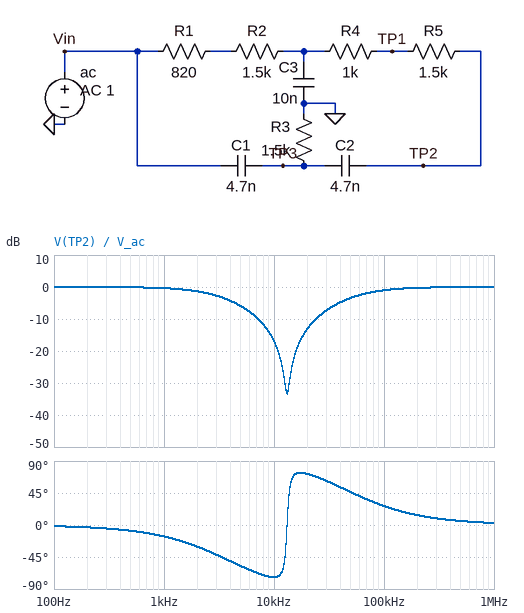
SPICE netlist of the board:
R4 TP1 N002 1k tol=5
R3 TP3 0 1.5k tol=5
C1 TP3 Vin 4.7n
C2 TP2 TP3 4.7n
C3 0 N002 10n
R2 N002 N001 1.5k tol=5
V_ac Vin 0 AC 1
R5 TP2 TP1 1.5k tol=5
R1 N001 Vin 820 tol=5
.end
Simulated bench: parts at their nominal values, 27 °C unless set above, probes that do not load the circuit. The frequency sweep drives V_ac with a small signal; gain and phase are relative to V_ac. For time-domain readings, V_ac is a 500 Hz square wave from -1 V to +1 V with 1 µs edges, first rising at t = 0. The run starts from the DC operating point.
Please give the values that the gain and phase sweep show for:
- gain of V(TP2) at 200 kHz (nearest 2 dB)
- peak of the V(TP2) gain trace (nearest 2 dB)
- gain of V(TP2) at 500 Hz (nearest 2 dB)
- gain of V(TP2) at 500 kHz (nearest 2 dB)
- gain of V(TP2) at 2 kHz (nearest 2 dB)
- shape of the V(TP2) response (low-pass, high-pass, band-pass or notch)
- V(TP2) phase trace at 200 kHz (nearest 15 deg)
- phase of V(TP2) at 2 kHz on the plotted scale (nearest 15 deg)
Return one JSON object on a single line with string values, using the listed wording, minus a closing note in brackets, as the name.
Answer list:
{"gain of V(TP2) at 200 kHz": "0 dB", "peak of the V(TP2) gain trace": "0 dB", "gain of V(TP2) at 500 Hz": "0 dB", "gain of V(TP2) at 500 kHz": "0 dB", "gain of V(TP2) at 2 kHz": "-2 dB", "shape of the V(TP2) response": "notch", "V(TP2) phase trace at 200 kHz": "15 deg", "phase of V(TP2) at 2 kHz on the plotted scale": "-30 deg"}
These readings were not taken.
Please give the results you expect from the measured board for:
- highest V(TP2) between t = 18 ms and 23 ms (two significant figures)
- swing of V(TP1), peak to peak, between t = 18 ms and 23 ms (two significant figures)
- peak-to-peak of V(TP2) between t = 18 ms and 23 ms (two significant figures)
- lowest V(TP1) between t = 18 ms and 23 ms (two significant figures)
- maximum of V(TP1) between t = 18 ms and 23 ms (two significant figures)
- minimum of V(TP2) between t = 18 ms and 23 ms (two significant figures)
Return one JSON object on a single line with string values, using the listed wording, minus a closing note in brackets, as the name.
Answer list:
{"highest V(TP2) between t = 18 ms and 23 ms": "1.0 V", "swing of V(TP1), peak to peak, between t = 18 ms and 23 ms": "2.0 V", "peak-to-peak of V(TP2) between t = 18 ms and 23 ms": "2.0 V", "lowest V(TP1) between t = 18 ms and 23 ms": "-1.0 V", "maximum of V(TP1) between t = 18 ms and 23 ms": "1.0 V", "minimum of V(TP2) between t = 18 ms and 23 ms": "-1.0 V"}
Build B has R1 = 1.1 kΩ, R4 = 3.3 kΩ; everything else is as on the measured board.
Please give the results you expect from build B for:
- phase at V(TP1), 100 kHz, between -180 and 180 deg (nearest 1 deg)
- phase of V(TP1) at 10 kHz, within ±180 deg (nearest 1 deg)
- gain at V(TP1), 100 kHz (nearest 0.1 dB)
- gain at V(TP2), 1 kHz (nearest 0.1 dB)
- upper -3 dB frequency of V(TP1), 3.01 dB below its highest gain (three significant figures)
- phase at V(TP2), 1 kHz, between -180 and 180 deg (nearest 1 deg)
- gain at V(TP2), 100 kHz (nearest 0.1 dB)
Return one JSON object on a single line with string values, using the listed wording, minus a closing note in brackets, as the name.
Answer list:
{"phase at V(TP1), 100 kHz, between -180 and 180 deg": "18 deg", "phase of V(TP1) at 10 kHz, within ±180 deg": "-48 deg", "gain at V(TP1), 100 kHz": "-3.8 dB", "gain at V(TP2), 1 kHz": "-0.6 dB", "upper -3 dB frequency of V(TP1), 3.01 dB below its highest gain": "2.67 kHz", "phase at V(TP2), 1 kHz, between -180 and 180 deg": "-21 deg", "gain at V(TP2), 100 kHz": "-0.5 dB"}
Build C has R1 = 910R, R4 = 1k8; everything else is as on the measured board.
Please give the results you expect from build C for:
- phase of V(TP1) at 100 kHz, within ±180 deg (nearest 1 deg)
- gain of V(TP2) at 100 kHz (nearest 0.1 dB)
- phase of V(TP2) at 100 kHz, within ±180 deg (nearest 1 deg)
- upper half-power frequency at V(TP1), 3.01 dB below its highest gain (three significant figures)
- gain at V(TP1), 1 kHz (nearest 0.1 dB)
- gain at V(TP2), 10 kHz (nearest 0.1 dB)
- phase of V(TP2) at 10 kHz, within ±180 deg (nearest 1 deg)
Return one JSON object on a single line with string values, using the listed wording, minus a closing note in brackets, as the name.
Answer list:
{"phase of V(TP1) at 100 kHz, within ±180 deg": "18 deg", "gain of V(TP2) at 100 kHz": "-0.8 dB", "phase of V(TP2) at 100 kHz, within ±180 deg": "24 deg", "upper half-power frequency at V(TP1), 3.01 dB below its highest gain": "3.19 kHz", "gain at V(TP1), 1 kHz": "-0.4 dB", "gain at V(TP2), 10 kHz": "-21.9 dB", "phase of V(TP2) at 10 kHz, within ±180 deg": "-84 deg"}
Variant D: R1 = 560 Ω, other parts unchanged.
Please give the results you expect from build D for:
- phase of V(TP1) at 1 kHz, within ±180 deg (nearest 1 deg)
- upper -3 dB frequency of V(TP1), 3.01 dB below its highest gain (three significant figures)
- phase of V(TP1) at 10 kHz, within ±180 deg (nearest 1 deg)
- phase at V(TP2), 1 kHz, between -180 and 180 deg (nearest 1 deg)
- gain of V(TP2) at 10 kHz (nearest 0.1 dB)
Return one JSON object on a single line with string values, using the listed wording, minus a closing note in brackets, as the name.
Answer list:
{"phase of V(TP1) at 1 kHz, within ±180 deg": "-12 deg", "upper -3 dB frequency of V(TP1), 3.01 dB below its highest gain": "3.90 kHz", "phase of V(TP1) at 10 kHz, within ±180 deg": "-48 deg", "phase at V(TP2), 1 kHz, between -180 and 180 deg": "-15 deg", "gain of V(TP2) at 10 kHz": "-15.2 dB"}
